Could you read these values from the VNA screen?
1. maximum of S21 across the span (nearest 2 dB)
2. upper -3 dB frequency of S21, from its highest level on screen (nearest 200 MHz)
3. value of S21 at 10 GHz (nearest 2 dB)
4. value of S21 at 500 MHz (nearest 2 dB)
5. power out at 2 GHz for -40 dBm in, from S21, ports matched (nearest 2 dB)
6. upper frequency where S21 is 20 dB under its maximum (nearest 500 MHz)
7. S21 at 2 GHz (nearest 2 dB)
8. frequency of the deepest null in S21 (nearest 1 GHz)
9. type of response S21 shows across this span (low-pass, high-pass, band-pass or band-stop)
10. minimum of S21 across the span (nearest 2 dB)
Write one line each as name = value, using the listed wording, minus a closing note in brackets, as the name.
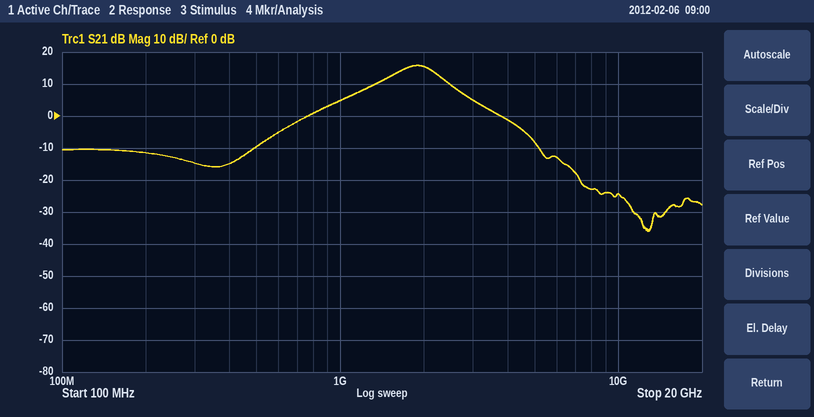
maximum of S21 across the span = 16 dB
upper -3 dB frequency of S21, from its highest level on screen = 2.2 GHz
value of S21 at 10 GHz = -24 dB
value of S21 at 500 MHz = -10 dB
power out at 2 GHz for -40 dBm in, from S21, ports matched = -24 dBm
upper frequency where S21 is 20 dB under its maximum = 4.5 GHz
S21 at 2 GHz = 16 dB
frequency of the deepest null in S21 = 13 GHz
type of response S21 shows across this span = band-pass
minimum of S21 across the span = -36 dB
